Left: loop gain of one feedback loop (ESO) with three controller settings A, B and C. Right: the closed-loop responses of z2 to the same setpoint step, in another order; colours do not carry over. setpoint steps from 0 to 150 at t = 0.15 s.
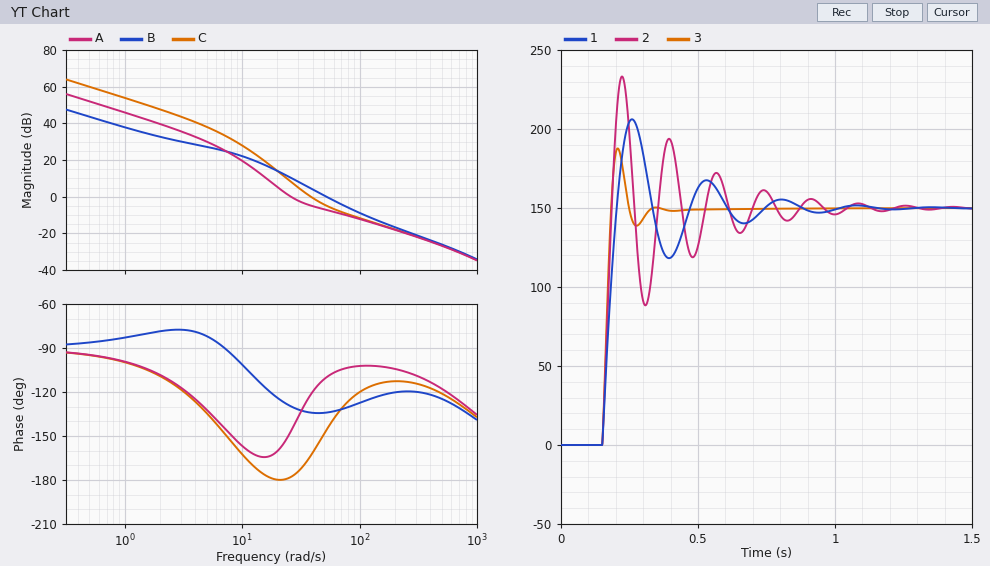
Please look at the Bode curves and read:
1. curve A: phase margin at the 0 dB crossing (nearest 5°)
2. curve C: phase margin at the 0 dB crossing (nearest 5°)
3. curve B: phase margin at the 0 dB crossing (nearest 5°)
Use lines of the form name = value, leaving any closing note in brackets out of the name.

curve A: phase margin at the 0 dB crossing = 35°
curve C: phase margin at the 0 dB crossing = 15°
curve B: phase margin at the 0 dB crossing = 45°
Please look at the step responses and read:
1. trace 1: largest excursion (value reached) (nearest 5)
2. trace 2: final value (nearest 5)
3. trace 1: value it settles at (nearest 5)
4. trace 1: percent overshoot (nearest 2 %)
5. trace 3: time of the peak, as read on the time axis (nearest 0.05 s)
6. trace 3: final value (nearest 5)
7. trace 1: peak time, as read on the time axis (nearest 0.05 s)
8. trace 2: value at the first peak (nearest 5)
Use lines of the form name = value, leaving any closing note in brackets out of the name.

trace 1: largest excursion (value reached) = 205
trace 2: final value = 150
trace 1: value it settles at = 150
trace 1: percent overshoot = 38 %
trace 3: time of the peak, as read on the time axis = 0.20 s
trace 3: final value = 150
trace 1: peak time, as read on the time axis = 0.25 s
trace 2: value at the first peak = 235
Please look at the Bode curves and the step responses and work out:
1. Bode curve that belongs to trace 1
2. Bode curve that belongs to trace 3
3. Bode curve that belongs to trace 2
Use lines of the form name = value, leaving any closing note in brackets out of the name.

Bode curve that belongs to trace 1 = A
Bode curve that belongs to trace 3 = B
Bode curve that belongs to trace 2 = C
